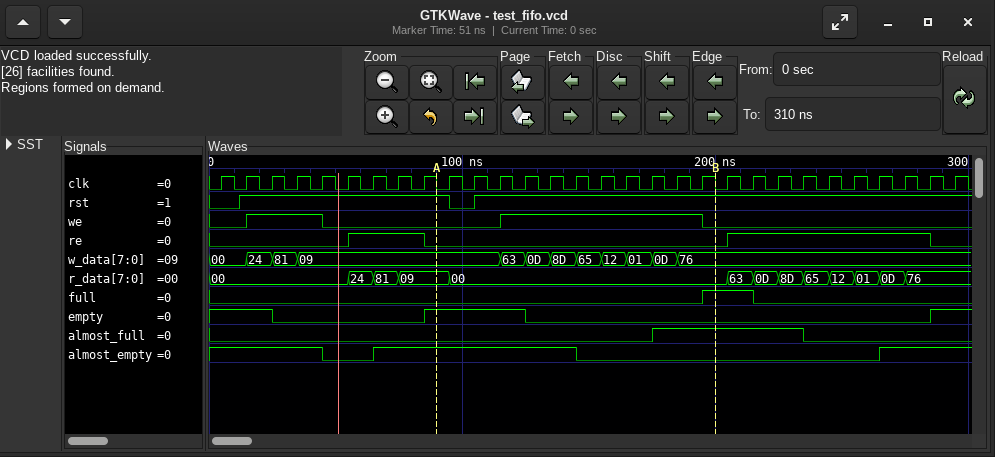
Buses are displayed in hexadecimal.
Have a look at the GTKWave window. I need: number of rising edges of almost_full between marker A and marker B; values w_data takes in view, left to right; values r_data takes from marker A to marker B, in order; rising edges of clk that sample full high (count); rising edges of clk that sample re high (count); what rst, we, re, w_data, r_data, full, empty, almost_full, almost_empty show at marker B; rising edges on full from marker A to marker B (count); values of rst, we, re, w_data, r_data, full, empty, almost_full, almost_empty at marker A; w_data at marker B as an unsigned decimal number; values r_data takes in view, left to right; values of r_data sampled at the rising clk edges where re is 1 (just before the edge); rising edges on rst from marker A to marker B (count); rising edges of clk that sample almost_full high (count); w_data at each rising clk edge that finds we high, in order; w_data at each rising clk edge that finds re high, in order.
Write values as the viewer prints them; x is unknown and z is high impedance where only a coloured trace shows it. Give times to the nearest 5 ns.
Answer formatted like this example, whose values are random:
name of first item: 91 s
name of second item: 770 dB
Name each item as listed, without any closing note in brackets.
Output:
number of rising edges of almost_full between marker A and marker B: 1
values w_data takes in view, left to right: 00, 24, 81, 09, 63, 0D, 8D, 65, 12, 01, 0D, 76
values r_data takes from marker A to marker B, in order: 09, 00
rising edges of clk that sample full high: 2
rising edges of clk that sample re high: 11
what rst, we, re, w_data, r_data, full, empty, almost_full, almost_empty show at marker B: rst=1, we=0, re=0, w_data=76, r_data=00, full=1, empty=0, almost_full=1, almost_empty=0
rising edges on full from marker A to marker B: 1
values of rst, we, re, w_data, r_data, full, empty, almost_full, almost_empty at marker A: rst=1, we=0, re=0, w_data=09, r_data=09, full=0, empty=1, almost_full=0, almost_empty=1
w_data at marker B as an unsigned decimal number: 118
values r_data takes in view, left to right: 00, 24, 81, 09, 00, 63, 0D, 8D, 65, 12, 01, 0D, 76
values of r_data sampled at the rising clk edges where re is 1: 24, 81, 09, 63, 0D, 8D, 65, 12, 01, 0D, 76
rising edges on rst from marker A to marker B: 1
rising edges of clk that sample almost_full high: 6
w_data at each rising clk edge that finds we high, in order: 24, 81, 09, 63, 0D, 8D, 65, 12, 01, 0D, 76
w_data at each rising clk edge that finds re high, in order: 09, 09, 09, 76, 76, 76, 76, 76, 76, 76, 76
